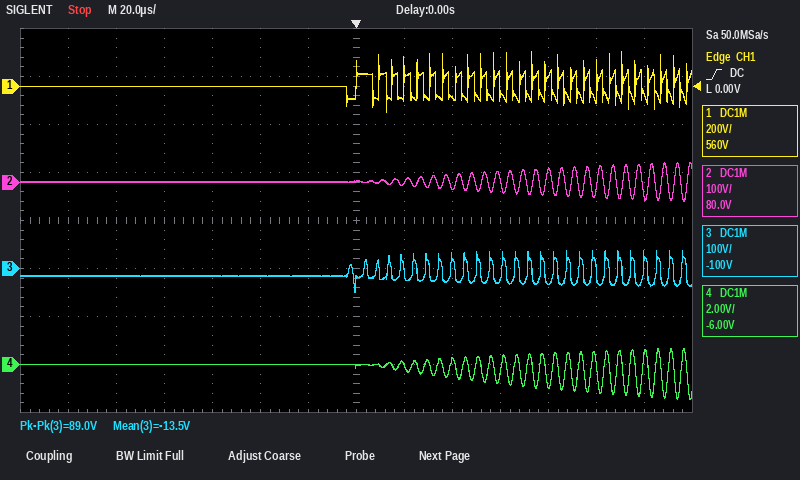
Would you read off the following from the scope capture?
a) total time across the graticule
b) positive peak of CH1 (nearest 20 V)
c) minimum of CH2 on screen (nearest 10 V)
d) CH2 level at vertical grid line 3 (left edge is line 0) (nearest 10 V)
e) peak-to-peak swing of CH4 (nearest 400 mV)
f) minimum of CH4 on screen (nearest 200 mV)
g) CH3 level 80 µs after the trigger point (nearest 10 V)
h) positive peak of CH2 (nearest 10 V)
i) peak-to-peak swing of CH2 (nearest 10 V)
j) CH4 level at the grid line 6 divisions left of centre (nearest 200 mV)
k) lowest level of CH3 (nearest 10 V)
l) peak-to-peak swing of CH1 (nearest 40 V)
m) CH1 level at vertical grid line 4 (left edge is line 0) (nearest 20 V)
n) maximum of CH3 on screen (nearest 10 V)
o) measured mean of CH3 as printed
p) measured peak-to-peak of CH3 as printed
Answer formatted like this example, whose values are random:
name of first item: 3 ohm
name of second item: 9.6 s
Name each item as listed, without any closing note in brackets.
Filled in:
total time across the graticule: 280 µs
positive peak of CH1: 140 V
minimum of CH2 on screen: -40 V
CH2 level at vertical grid line 3 (left edge is line 0): 0 V
peak-to-peak swing of CH4: 2.0 V
minimum of CH4 on screen: -1.4 V
CH3 level 80 µs after the trigger point: -30 V
positive peak of CH2: 40 V
peak-to-peak swing of CH2: 80 V
CH4 level at the grid line 6 divisions left of centre: 0.0 V
lowest level of CH3: -50 V
peak-to-peak swing of CH1: 240 V
CH1 level at vertical grid line 4 (left edge is line 0): 0 V
maximum of CH3 on screen: 40 V
measured mean of CH3 as printed: -13.5 V
measured peak-to-peak of CH3 as printed: 89.0 V
